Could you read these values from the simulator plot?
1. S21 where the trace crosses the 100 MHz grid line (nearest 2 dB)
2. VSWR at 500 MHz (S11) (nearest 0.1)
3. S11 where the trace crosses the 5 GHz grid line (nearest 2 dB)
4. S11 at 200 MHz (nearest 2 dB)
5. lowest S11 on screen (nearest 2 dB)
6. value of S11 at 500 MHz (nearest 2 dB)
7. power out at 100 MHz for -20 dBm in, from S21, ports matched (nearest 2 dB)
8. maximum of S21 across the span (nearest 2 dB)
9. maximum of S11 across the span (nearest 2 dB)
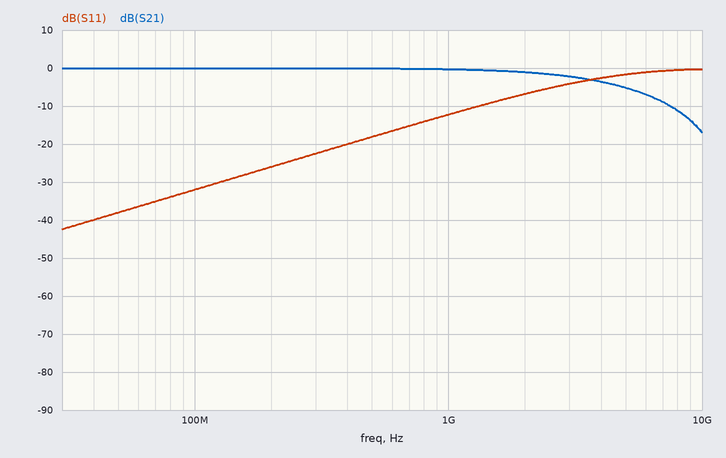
0 dB
1.3
-2 dB
-26 dB
-42 dB
-18 dB
-20 dBm
0 dB
0 dB
